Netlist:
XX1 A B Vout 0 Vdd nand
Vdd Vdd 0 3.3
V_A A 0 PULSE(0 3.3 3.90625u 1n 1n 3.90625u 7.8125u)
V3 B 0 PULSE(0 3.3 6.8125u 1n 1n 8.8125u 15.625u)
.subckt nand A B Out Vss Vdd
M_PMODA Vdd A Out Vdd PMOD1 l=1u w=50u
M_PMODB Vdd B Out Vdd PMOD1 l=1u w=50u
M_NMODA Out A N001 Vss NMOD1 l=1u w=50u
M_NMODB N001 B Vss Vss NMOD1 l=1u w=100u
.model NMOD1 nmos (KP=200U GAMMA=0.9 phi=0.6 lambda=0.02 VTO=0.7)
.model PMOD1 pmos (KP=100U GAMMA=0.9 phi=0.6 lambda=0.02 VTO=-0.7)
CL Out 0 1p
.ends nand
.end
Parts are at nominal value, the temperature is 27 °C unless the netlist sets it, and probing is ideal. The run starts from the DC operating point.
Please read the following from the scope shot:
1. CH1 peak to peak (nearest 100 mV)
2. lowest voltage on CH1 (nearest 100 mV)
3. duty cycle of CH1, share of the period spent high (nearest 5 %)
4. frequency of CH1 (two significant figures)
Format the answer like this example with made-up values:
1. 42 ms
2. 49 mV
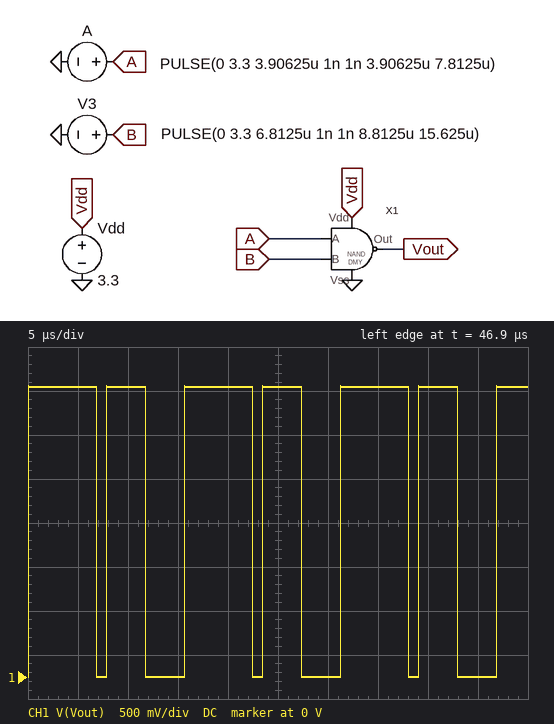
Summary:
1. 3.3 V
2. 0 V
3. 70 %
4. 130 kHz
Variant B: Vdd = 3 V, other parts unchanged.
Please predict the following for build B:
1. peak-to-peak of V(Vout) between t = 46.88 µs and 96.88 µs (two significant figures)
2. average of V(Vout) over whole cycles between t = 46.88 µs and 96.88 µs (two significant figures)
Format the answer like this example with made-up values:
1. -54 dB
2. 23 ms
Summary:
1. 3.0 V
2. 2.1 V
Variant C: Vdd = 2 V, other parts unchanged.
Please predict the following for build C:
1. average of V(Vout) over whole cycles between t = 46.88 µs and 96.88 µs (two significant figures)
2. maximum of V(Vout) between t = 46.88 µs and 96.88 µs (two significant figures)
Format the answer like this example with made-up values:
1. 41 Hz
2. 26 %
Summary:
1. 1.4 V
2. 2.0 V
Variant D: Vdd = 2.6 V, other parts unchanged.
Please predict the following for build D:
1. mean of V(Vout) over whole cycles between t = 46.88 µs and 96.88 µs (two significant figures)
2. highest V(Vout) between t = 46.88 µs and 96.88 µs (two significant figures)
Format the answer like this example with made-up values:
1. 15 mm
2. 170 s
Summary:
1. 1.8 V
2. 2.6 V
